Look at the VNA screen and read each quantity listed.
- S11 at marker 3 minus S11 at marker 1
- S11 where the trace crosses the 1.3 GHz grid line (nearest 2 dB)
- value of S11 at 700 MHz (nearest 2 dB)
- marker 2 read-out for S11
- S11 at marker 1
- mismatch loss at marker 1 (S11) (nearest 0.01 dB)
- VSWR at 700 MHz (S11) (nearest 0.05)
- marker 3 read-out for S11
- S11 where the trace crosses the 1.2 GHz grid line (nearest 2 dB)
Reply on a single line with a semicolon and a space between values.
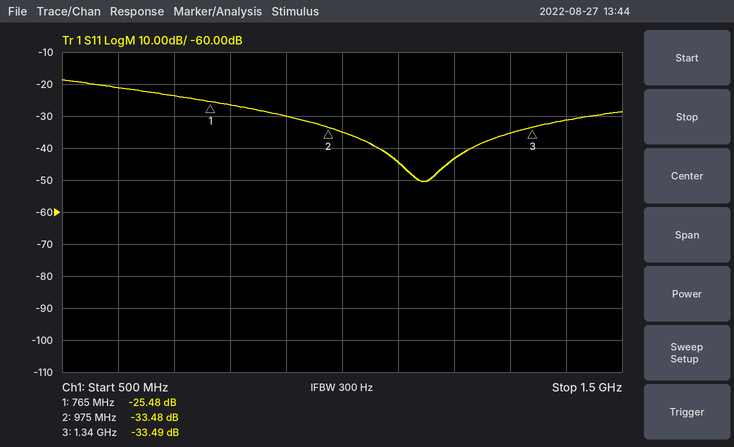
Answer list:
-8.01 dB; -36 dB; -24 dB; -33.48 dB; -25.48 dB; 0.01 dB; 1.15; -33.49 dB; -44 dB
